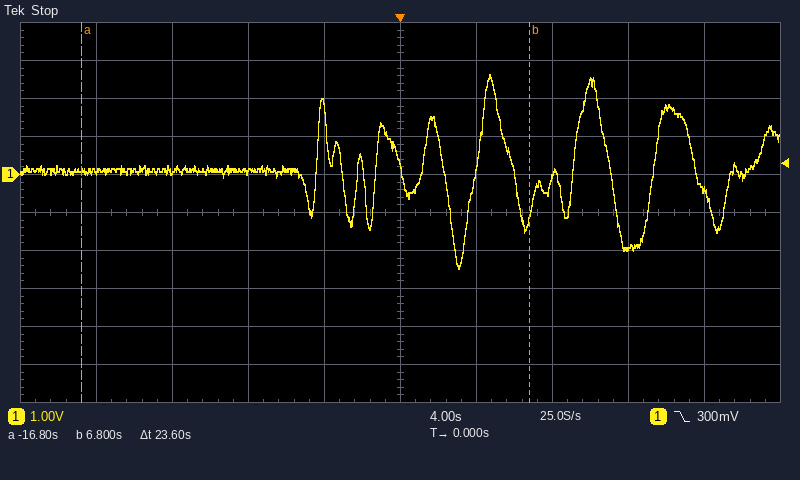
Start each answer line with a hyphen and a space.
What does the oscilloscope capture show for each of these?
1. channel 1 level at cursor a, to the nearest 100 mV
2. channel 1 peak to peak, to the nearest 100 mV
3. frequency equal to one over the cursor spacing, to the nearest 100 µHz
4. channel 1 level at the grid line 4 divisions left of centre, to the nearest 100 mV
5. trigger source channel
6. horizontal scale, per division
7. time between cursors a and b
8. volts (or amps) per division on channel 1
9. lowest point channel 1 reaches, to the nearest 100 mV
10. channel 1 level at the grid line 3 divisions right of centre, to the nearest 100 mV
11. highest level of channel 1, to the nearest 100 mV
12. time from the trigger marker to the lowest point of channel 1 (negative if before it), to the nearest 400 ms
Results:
- 100 mV
- 5.1 V
- 42.4 mHz
- 100 mV
- channel 1
- 4 s
- 23.6 s
- 1 V
- -2.5 V
- -1.9 V
- 2.6 V
- +3.2 s
